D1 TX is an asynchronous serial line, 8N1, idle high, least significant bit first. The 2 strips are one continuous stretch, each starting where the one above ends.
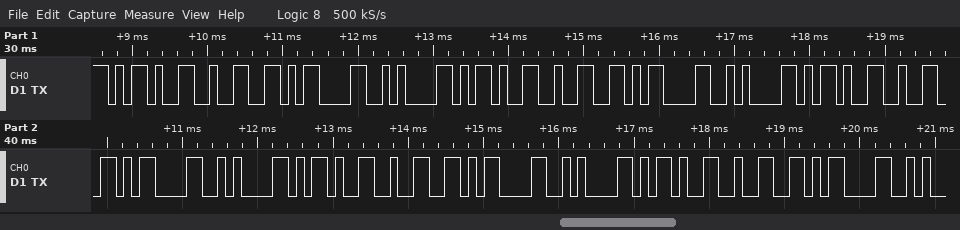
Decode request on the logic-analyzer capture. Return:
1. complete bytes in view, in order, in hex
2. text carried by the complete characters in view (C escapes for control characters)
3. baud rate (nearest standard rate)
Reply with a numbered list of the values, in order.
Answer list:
1. 2D 32 0D 0A 2D 32 0D 0A 2D 32 0D 0A 2D 32 0D 0A 2D 32 0D
2. "-2\r\n-2\r\n-2\r\n-2\r\n-2\r"
3. 9600 baud
